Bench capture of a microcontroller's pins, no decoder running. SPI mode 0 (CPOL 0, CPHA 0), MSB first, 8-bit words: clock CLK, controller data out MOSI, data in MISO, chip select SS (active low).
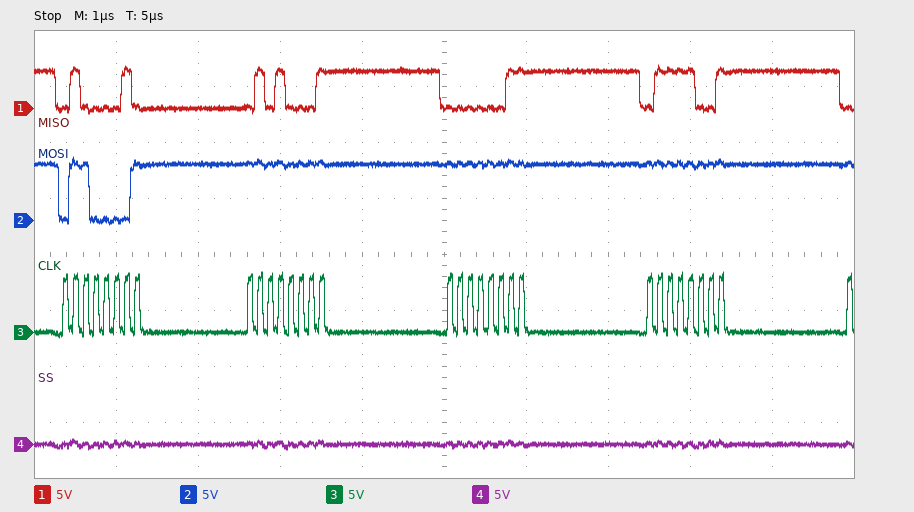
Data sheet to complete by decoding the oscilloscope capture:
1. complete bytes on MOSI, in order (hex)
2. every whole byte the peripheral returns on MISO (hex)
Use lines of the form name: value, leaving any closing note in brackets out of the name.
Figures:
complete bytes on MOSI, in order: 61 FF FF FF
every whole byte the peripheral returns on MISO: 42 51 03 79
